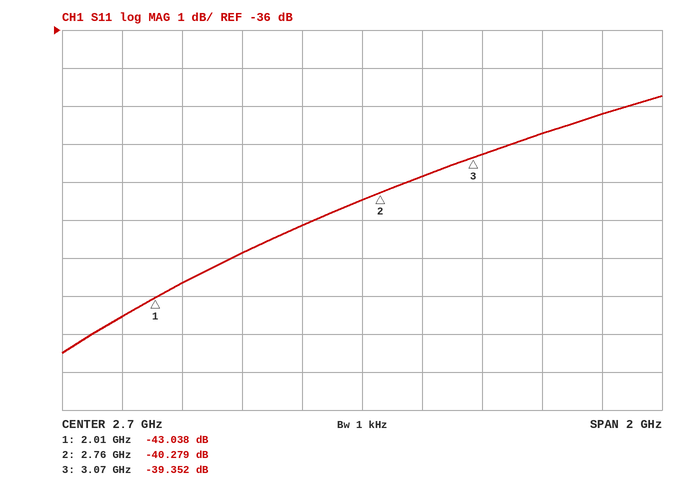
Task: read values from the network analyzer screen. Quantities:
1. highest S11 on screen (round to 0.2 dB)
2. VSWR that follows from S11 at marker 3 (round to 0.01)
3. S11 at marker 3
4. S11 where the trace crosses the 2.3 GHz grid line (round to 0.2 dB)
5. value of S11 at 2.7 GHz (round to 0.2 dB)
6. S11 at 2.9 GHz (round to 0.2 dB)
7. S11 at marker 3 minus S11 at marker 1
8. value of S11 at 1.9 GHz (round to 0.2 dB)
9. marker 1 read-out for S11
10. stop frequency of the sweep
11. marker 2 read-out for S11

-37.8 dB
1.02
-39.352 dB
-41.8 dB
-40.4 dB
-39.8 dB
3.686 dB
-43.6 dB
-43.038 dB
3.7 GHz
-40.279 dB
